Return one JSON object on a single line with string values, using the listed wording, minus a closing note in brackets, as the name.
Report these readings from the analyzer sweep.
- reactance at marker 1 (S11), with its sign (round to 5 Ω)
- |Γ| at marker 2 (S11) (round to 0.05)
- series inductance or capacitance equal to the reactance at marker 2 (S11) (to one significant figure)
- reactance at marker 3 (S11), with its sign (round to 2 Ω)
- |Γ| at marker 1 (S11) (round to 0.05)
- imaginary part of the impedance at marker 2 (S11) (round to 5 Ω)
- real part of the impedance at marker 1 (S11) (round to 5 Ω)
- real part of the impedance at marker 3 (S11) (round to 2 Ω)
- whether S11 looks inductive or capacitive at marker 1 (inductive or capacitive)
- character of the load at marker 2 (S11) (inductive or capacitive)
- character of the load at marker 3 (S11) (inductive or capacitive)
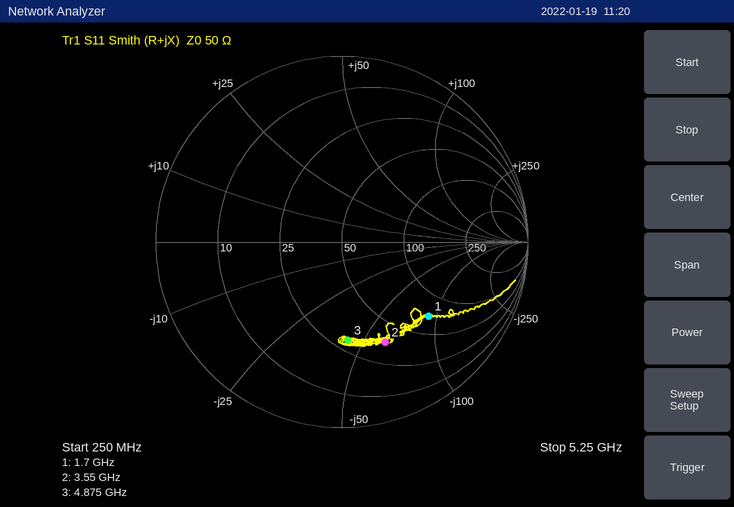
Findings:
{"reactance at marker 1 (S11), with its sign": "-90 Ω", "|Γ| at marker 2 (S11)": "0.60", "series inductance or capacitance equal to the reactance at marker 2 (S11)": "700 fF", "reactance at marker 3 (S11), with its sign": "-44 Ω", "|Γ| at marker 1 (S11)": "0.60", "imaginary part of the impedance at marker 2 (S11)": "-60 Ω", "real part of the impedance at marker 1 (S11)": "70 Ω", "real part of the impedance at marker 3 (S11)": "30 Ω", "whether S11 looks inductive or capacitive at marker 1": "capacitive", "character of the load at marker 2 (S11)": "capacitive", "character of the load at marker 3 (S11)": "capacitive"}
